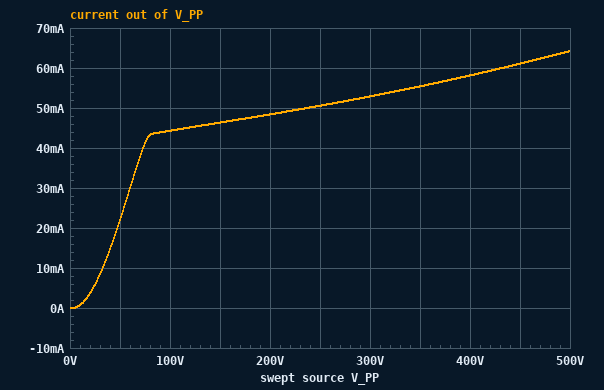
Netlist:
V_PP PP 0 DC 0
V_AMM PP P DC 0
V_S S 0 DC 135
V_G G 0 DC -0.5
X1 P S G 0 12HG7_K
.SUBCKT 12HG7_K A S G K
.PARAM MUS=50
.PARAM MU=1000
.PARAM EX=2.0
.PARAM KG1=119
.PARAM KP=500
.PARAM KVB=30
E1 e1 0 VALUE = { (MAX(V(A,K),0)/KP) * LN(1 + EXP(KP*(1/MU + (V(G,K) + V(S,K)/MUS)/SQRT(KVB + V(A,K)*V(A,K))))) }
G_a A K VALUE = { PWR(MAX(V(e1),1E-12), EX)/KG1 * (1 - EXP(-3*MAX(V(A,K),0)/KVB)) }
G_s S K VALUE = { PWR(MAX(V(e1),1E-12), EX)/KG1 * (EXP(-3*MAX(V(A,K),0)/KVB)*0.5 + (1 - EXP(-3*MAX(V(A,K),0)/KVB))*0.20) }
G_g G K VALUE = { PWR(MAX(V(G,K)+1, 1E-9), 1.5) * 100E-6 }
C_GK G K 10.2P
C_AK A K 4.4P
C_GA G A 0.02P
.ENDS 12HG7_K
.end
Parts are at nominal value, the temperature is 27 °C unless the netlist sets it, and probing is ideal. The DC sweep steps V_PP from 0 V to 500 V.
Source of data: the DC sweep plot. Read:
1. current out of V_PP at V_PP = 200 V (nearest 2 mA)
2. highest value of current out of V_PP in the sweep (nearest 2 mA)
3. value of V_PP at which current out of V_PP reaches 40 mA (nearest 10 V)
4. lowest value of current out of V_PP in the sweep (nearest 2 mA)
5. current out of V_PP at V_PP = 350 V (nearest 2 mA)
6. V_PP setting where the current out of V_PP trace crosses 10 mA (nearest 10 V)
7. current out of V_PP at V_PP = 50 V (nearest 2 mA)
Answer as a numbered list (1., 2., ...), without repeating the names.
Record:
1. 48 mA
2. 64 mA
3. 70 V
4. 0 A
5. 56 mA
6. 30 V
7. 22 mA
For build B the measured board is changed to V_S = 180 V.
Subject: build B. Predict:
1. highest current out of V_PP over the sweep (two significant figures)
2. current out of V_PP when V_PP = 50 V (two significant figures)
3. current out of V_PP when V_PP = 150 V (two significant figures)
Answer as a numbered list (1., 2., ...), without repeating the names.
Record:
1. 110 mA
2. 24 mA
3. 89 mA
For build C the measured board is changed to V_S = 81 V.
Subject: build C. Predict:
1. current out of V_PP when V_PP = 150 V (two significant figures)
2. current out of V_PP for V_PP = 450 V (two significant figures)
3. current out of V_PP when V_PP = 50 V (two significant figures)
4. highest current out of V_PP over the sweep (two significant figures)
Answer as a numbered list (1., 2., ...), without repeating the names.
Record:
1. 14 mA
2. 25 mA
3. 11 mA
4. 27 mA
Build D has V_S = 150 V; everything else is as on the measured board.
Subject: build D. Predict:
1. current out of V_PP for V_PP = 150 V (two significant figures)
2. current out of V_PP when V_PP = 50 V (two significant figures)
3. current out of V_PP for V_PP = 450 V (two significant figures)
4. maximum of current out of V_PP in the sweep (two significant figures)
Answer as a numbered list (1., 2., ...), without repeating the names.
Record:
1. 59 mA
2. 23 mA
3. 75 mA
4. 78 mA
